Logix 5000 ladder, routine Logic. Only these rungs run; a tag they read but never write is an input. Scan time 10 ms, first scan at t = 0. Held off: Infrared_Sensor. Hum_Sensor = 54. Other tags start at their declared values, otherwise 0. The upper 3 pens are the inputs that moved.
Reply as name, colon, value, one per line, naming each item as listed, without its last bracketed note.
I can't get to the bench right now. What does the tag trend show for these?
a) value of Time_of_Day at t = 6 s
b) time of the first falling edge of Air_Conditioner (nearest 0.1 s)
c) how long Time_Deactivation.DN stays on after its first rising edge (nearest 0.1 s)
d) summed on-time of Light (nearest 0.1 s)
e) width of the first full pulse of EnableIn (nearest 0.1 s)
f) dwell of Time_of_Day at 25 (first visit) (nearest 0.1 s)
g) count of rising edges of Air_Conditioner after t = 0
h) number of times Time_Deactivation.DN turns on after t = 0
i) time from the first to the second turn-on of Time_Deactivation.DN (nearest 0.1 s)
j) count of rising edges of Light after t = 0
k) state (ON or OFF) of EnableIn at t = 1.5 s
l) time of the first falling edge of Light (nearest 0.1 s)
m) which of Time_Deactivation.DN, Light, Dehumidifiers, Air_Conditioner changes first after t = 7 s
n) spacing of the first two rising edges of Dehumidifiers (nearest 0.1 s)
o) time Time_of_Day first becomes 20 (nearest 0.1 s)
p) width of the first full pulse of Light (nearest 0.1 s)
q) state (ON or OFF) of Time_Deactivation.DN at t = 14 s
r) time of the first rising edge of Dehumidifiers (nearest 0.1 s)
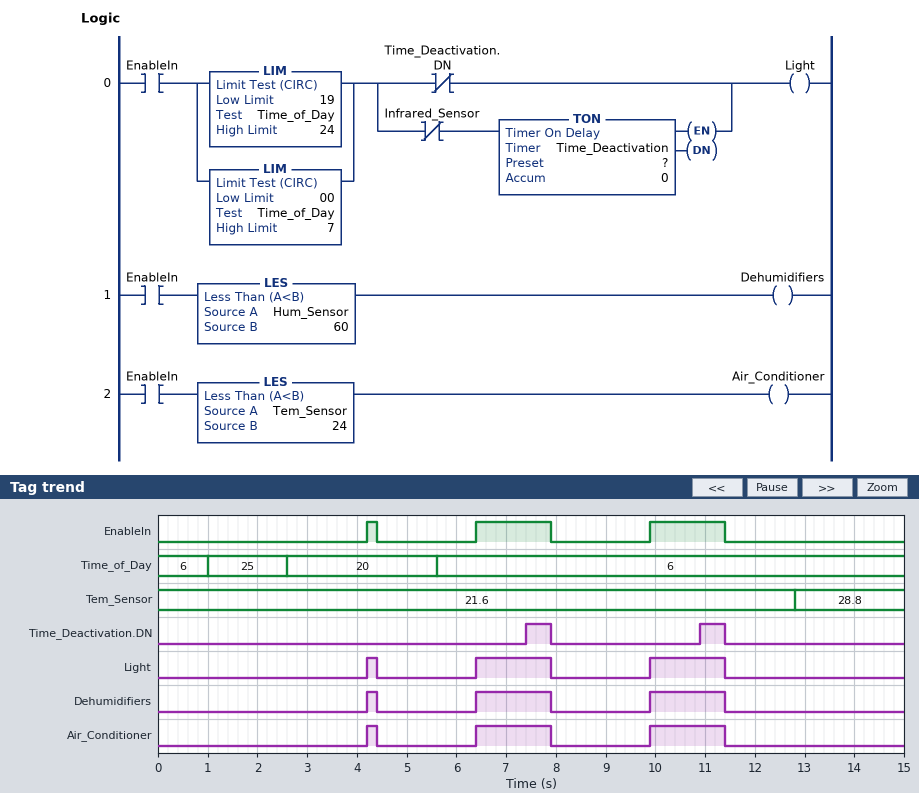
value of Time_of_Day at t = 6 s: 6
time of the first falling edge of Air_Conditioner: 4.4 s
how long Time_Deactivation.DN stays on after its first rising edge: 0.5 s
summed on-time of Light: 3.2 s
width of the first full pulse of EnableIn: 0.2 s
dwell of Time_of_Day at 25 (first visit): 1.6 s
count of rising edges of Air_Conditioner after t = 0: 3
number of times Time_Deactivation.DN turns on after t = 0: 2
time from the first to the second turn-on of Time_Deactivation.DN: 3.5 s
count of rising edges of Light after t = 0: 3
state (ON or OFF) of EnableIn at t = 1.5 s: OFF
time of the first falling edge of Light: 4.4 s
which of Time_Deactivation.DN, Light, Dehumidifiers, Air_Conditioner changes first after t = 7 s: Time_Deactivation.DN
spacing of the first two rising edges of Dehumidifiers: 2.2 s
time Time_of_Day first becomes 20: 2.6 s
width of the first full pulse of Light: 0.2 s
state (ON or OFF) of Time_Deactivation.DN at t = 14 s: OFF
time of the first rising edge of Dehumidifiers: 4.2 s
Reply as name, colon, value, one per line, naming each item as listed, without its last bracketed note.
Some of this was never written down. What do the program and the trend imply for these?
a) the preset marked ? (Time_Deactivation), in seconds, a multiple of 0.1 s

the preset marked ? (Time_Deactivation), in seconds, a multiple of 0.1 s: 1.0 s
